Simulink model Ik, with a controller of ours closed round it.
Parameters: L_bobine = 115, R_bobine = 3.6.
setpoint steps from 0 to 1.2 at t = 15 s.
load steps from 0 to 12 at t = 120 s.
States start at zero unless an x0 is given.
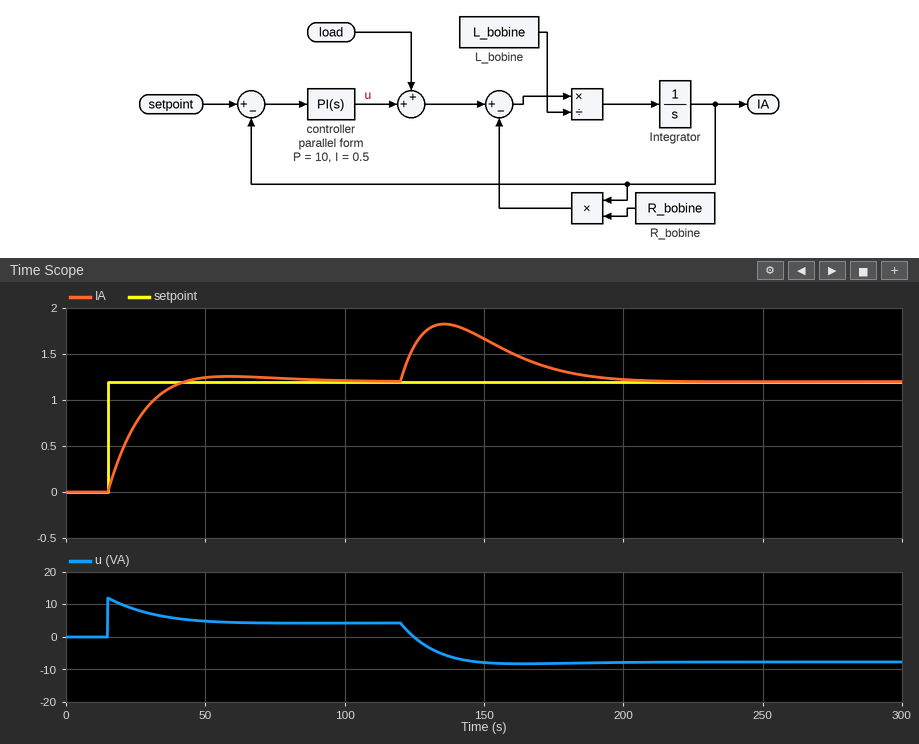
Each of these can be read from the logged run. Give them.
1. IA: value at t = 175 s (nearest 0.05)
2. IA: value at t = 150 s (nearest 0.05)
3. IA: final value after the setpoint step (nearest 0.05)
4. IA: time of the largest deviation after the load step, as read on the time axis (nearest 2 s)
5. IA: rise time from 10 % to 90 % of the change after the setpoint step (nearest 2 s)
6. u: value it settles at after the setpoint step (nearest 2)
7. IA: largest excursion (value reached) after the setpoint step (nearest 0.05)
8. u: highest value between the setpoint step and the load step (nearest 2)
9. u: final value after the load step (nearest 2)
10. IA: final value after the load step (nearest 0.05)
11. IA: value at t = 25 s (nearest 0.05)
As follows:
1.35
1.65
1.20
136 s
18 s
4
1.25
12
-8
1.20
0.75
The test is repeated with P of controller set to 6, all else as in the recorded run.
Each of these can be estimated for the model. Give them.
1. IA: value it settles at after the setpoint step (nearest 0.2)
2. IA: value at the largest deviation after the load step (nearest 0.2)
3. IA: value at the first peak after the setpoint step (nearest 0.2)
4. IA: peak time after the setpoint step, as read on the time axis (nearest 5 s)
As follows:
1.2
2.0
1.4
60 s
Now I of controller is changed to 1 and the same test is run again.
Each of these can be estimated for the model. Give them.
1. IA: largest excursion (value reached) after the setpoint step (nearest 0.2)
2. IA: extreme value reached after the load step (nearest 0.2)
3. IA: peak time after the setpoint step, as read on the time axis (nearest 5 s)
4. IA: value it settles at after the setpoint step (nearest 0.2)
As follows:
1.4
1.8
45 s
1.2
